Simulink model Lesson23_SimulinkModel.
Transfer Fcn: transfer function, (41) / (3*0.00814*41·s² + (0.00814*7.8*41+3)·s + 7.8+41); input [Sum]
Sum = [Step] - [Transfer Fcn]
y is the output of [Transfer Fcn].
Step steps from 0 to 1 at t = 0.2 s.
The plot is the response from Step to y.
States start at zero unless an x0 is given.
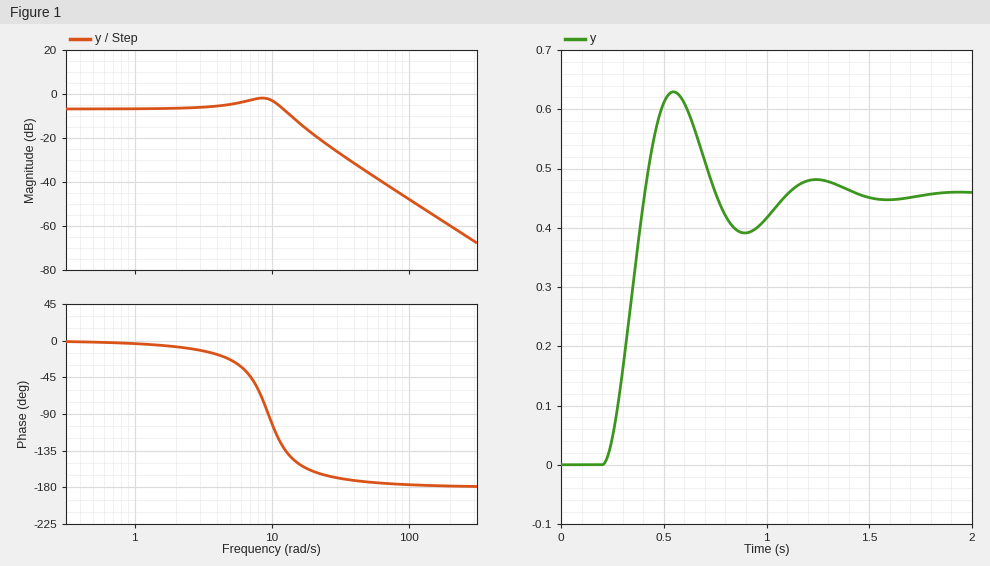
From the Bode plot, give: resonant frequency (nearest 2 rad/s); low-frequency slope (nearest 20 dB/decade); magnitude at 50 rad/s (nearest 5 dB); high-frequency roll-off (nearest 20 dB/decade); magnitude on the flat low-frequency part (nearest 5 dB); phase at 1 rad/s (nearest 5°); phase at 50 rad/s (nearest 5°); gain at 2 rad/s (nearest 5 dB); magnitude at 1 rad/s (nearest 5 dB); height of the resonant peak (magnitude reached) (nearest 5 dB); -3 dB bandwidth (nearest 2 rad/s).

8 rad/s
0 dB/decade
-35 dB
-40 dB/decade
-5 dB
-5°
-175°
-5 dB
-5 dB
0 dB
14 rad/s
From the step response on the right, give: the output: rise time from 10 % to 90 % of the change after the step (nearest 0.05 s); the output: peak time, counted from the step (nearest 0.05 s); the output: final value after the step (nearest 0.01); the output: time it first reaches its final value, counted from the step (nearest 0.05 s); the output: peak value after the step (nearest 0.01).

0.15 s
0.35 s
0.46
0.20 s
0.63
